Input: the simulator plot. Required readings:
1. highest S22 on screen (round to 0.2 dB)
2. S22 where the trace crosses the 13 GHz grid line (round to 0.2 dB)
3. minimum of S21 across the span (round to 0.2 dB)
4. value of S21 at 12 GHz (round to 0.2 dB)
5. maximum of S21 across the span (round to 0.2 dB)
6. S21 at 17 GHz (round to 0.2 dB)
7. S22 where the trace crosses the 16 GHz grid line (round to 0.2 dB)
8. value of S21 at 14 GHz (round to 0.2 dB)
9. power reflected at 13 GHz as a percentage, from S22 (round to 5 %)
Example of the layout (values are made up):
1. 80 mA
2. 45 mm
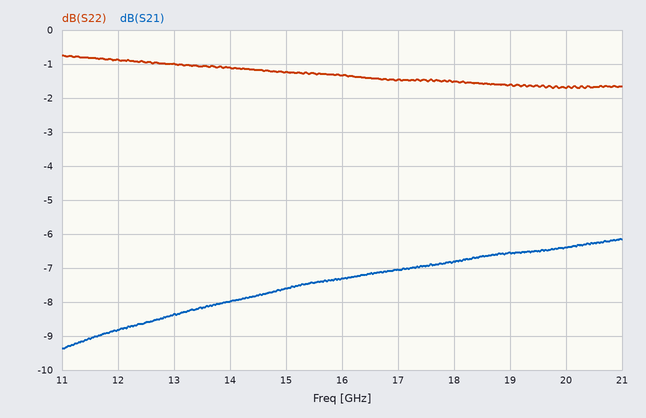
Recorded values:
1. -0.8 dB
2. -1.0 dB
3. -9.4 dB
4. -8.8 dB
5. -6.2 dB
6. -7.0 dB
7. -1.4 dB
8. -8.0 dB
9. 80 %
